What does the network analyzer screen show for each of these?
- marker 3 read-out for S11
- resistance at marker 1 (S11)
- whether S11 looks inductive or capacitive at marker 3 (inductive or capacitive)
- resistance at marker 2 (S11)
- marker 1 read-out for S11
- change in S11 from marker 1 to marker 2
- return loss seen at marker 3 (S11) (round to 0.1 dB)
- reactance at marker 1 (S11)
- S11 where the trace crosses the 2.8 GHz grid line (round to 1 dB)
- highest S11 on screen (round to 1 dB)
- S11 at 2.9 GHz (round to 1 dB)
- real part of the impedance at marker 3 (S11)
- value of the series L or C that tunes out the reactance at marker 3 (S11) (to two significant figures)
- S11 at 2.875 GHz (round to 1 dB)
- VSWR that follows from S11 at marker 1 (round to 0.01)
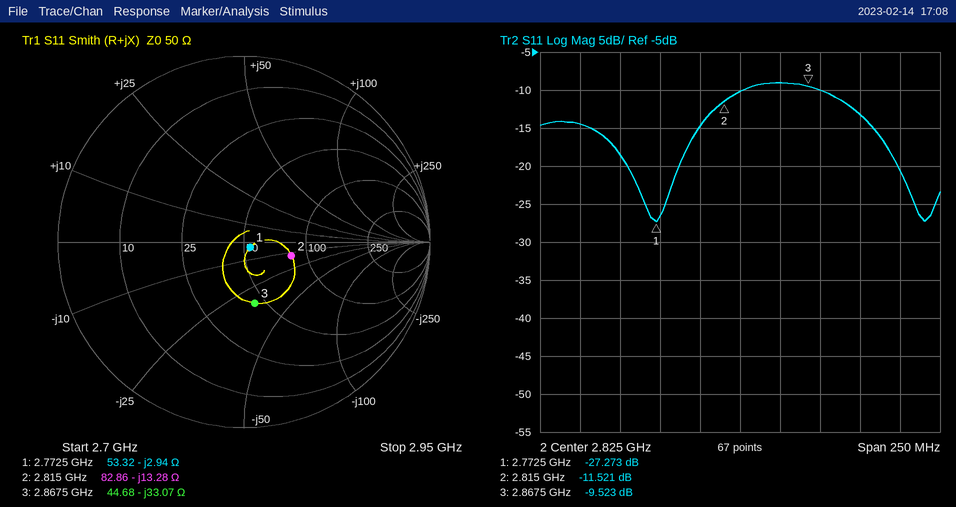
-9.523 dB
53.32 Ω
capacitive
82.86 Ω
-27.273 dB
15.752 dB
9.5 dB
-2.94 Ω
-15 dB
-9 dB
-13 dB
44.68 Ω
1.8 nH
-10 dB
1.09
